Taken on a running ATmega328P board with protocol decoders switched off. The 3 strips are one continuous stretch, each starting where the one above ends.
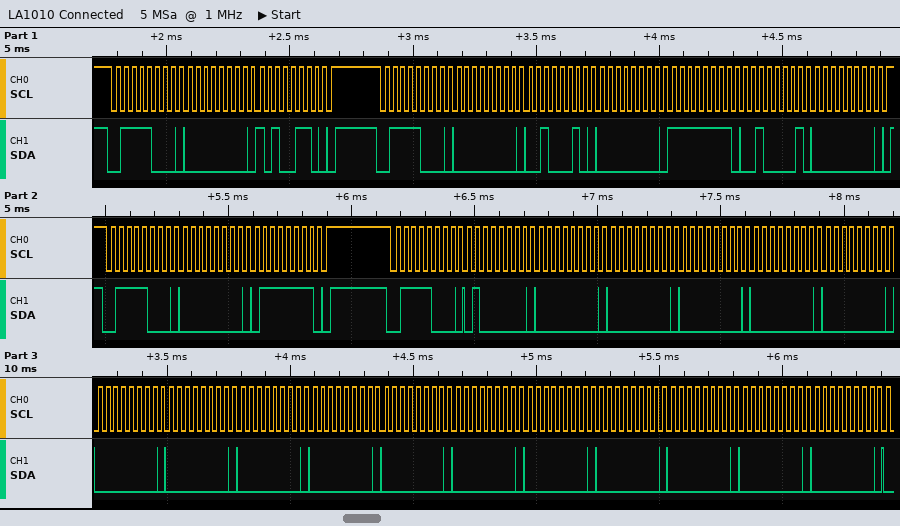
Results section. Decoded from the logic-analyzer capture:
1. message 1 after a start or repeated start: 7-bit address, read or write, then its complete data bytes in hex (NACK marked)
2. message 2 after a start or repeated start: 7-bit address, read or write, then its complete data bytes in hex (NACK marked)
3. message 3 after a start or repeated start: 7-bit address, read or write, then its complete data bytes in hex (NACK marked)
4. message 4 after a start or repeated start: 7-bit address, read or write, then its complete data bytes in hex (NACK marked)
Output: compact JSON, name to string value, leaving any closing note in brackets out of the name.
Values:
{"message 1 after a start or repeated start: 7-bit address, read or write, then its complete data bytes in hex": "0x3C write: 00 A6", "message 2 after a start or repeated start: 7-bit address, read or write, then its complete data bytes in hex": "0x3C write: 00 22 00 FF 21 00", "message 3 after a start or repeated start: 7-bit address, read or write, then its complete data bytes in hex": "0x3C write: 00 7F", "message 4 after a start or repeated start: 7-bit address, read or write, then its complete data bytes in hex": "0x3C write: 40 00 00 00 00 00 00 00 00 00 00 00 00 00 00 00 00"}
